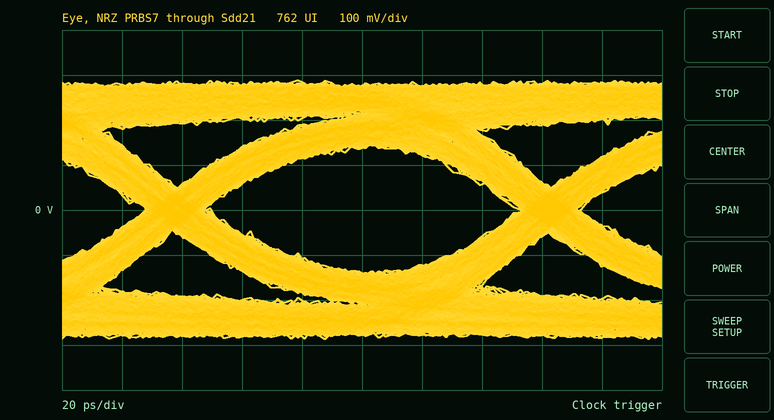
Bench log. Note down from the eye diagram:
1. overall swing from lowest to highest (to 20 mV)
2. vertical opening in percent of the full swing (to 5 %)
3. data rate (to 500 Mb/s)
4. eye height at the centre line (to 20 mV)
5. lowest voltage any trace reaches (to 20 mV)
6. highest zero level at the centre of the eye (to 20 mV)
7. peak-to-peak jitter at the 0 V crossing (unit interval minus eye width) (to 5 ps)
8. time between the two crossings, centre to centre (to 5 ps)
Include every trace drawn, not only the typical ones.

580 mV
50 %
8.0 Gb/s
280 mV
-280 mV
-140 mV
20 ps
125 ps
